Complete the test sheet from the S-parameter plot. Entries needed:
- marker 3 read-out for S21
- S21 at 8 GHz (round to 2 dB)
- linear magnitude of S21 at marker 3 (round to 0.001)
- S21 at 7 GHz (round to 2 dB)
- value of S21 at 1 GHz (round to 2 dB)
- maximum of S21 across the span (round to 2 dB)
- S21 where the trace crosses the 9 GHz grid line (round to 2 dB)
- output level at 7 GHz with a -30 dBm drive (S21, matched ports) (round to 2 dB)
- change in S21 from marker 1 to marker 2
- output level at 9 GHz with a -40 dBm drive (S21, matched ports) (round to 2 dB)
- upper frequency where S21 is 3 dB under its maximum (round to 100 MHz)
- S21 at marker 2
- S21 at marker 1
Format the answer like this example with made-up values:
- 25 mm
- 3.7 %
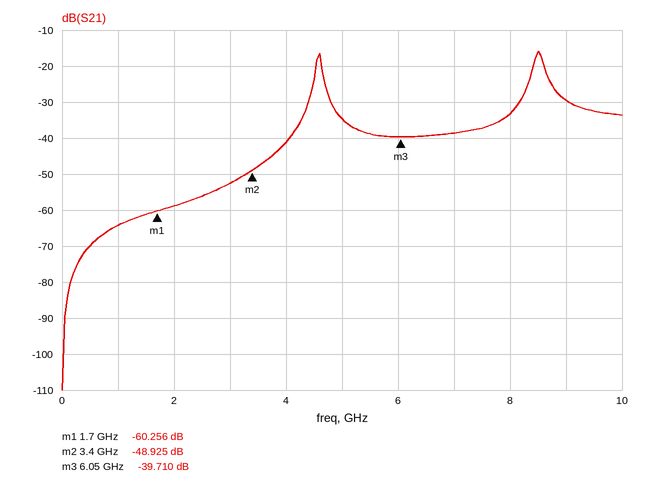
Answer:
- -39.710 dB
- -34 dB
- 0.010
- -38 dB
- -64 dB
- -16 dB
- -30 dB
- -68 dBm
- 11.331 dB
- -70 dBm
- 8.6 GHz
- -48.925 dB
- -60.256 dB
